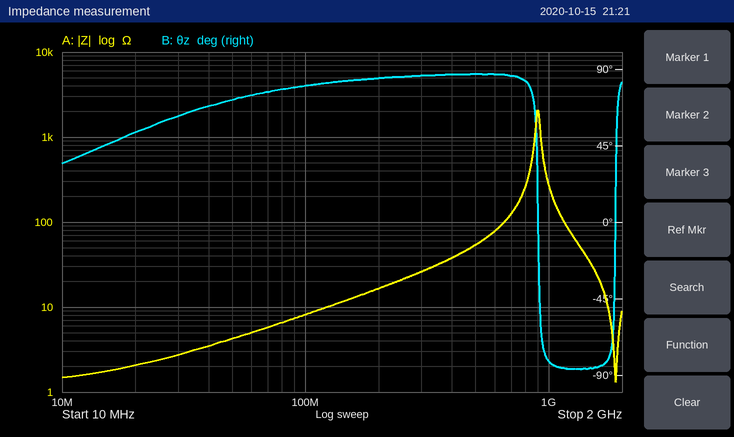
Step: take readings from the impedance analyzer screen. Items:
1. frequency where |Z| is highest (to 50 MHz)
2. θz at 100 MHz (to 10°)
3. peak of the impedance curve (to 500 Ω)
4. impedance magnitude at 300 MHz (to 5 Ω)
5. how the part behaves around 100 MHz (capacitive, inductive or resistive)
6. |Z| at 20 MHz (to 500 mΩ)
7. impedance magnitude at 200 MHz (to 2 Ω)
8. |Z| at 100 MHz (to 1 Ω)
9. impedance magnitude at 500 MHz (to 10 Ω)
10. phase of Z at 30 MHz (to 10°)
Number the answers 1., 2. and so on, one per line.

1. 900 MHz
2. 80°
3. 2.0 kΩ
4. 25 Ω
5. inductive
6. 2.0 Ω
7. 16 Ω
8. 8 Ω
9. 50 Ω
10. 60°
